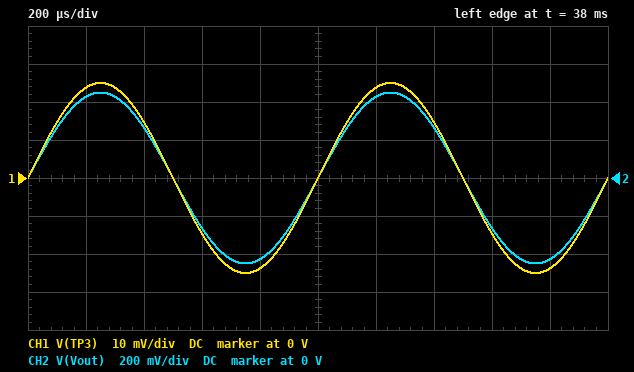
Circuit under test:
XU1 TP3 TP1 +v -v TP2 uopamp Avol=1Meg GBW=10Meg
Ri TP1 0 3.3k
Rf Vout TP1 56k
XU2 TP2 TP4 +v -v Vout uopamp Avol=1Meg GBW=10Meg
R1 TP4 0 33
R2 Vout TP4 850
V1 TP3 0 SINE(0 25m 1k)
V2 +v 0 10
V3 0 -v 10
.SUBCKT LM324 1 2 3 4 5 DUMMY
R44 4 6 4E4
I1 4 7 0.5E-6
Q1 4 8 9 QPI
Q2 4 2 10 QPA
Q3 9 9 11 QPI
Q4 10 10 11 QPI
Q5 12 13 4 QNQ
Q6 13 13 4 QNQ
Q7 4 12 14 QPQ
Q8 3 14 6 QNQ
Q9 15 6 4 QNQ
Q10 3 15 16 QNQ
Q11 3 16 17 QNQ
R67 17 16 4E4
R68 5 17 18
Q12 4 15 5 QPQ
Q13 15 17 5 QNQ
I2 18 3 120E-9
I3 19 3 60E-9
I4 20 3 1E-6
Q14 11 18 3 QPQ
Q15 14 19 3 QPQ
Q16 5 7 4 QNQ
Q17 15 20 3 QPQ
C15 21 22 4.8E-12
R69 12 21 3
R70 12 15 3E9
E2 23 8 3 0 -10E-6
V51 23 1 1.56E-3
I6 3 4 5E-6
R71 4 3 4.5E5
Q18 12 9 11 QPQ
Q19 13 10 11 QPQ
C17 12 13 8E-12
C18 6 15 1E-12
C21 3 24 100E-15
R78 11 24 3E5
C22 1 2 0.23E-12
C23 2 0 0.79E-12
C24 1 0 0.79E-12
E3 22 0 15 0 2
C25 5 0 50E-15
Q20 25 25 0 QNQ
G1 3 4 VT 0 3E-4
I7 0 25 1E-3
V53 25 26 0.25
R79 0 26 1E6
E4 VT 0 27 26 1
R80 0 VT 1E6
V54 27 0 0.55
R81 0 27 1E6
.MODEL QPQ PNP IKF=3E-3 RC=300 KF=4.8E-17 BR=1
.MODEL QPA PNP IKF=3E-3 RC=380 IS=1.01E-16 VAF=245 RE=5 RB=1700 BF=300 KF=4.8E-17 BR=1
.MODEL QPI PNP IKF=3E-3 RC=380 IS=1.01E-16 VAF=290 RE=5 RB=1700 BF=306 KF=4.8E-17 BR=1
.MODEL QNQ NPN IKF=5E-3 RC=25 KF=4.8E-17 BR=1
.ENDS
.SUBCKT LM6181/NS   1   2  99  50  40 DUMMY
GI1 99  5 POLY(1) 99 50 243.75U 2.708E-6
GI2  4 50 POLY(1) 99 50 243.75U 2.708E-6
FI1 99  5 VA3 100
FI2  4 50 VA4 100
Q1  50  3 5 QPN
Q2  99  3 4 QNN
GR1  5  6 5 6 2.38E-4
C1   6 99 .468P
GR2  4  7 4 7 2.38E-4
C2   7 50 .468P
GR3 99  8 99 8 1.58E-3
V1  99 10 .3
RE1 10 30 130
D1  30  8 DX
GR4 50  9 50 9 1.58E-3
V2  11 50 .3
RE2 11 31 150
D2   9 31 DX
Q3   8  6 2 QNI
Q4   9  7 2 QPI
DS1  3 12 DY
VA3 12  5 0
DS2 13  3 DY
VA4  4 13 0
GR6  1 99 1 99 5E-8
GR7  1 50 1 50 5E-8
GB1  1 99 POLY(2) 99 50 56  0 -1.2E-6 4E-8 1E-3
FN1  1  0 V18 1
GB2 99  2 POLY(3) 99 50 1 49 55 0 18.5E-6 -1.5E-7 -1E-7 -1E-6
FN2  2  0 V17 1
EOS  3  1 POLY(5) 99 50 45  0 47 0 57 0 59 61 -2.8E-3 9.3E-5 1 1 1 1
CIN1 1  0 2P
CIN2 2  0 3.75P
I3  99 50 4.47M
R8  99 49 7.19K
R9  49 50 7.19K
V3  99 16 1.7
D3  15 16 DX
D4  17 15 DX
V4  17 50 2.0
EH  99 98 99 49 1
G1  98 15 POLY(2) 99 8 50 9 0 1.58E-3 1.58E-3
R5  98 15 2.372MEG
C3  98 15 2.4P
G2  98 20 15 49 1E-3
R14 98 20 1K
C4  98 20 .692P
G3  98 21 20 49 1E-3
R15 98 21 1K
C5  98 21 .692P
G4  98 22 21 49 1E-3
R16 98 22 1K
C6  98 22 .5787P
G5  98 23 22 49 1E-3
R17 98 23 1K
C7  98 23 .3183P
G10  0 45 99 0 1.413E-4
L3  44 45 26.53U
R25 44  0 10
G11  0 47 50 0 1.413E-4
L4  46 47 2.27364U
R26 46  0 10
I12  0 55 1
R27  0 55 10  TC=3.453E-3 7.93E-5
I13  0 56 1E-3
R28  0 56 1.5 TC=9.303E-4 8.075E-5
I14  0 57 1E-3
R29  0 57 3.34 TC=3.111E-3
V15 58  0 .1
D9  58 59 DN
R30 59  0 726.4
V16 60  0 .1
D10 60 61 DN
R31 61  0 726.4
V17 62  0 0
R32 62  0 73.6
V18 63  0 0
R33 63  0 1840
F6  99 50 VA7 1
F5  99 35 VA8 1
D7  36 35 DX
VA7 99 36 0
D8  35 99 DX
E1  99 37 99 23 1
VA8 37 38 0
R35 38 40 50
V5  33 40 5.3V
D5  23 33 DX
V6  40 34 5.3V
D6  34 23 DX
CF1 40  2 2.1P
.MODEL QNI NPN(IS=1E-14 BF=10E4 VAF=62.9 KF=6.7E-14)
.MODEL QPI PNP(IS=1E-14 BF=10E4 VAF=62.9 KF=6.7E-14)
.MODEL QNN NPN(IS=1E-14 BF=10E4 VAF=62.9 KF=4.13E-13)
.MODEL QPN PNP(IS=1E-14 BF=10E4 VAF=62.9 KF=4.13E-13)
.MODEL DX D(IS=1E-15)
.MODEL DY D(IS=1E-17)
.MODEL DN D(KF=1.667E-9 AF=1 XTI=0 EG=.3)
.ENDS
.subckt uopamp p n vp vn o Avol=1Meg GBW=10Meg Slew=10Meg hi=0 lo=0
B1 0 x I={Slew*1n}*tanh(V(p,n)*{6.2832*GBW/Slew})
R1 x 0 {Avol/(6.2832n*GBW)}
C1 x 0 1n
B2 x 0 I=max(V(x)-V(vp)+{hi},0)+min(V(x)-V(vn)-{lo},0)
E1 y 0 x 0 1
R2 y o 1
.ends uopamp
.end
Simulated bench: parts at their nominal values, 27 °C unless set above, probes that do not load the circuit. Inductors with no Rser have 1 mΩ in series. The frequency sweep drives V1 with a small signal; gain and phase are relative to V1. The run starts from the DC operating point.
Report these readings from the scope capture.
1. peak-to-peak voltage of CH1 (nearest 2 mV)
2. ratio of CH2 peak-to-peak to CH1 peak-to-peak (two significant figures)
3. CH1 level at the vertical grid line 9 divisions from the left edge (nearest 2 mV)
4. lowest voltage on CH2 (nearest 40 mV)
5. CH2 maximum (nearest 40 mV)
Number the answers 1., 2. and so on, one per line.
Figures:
1. 50 mV
2. 18
3. -24 mV
4. -440 mV
5. 440 mV
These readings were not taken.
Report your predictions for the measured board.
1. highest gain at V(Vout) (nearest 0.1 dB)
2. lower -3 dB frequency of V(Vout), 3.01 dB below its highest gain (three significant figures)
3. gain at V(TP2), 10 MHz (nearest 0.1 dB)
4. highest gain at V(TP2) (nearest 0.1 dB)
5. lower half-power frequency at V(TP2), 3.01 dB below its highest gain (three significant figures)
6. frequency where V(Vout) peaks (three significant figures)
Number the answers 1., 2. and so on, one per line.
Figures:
1. 41.1 dB
2. 2.15 MHz
3. 0.5 dB
4. 28.7 dB
5. 2.18 MHz
6. 2.34 MHz
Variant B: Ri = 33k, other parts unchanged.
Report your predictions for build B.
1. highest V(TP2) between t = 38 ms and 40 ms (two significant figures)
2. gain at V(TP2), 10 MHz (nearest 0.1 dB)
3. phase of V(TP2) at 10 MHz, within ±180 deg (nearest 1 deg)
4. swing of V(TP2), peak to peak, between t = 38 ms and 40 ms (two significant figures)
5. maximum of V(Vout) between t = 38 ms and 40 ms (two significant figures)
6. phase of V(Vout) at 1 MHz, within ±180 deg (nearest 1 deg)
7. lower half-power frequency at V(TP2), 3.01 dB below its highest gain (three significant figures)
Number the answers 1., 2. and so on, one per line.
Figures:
1. 2.5 mV
2. 4.0 dB
3. -89 deg
4. 5.0 mV
5. 67 mV
6. -1 deg
7. 5.90 MHz
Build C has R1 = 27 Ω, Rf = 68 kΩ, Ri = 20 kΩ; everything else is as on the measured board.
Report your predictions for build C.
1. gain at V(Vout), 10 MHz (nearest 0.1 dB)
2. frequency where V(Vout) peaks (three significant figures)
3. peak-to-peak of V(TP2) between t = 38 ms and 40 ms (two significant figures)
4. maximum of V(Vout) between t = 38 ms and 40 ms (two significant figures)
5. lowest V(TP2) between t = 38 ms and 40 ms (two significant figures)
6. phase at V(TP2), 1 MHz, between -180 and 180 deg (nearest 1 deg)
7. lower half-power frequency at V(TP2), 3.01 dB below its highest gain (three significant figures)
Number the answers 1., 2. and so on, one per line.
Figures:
1. 2.2 dB
2. 4.76 MHz
3. 6.8 mV
4. 110 mV
5. -3.4 mV
6. 72 deg
7. 4.61 MHz
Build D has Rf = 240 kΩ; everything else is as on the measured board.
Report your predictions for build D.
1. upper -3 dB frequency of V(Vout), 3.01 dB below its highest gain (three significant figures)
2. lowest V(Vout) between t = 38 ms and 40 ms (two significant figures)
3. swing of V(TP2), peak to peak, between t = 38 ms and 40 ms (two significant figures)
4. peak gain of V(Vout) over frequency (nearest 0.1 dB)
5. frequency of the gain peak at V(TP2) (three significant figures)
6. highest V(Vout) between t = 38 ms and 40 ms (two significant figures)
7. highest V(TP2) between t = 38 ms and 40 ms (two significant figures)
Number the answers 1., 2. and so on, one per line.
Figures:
1. 1.31 MHz
2. -1.8 V
3. 140 mV
4. 47.3 dB
5. 1.16 MHz
6. 1.8 V
7. 69 mV
